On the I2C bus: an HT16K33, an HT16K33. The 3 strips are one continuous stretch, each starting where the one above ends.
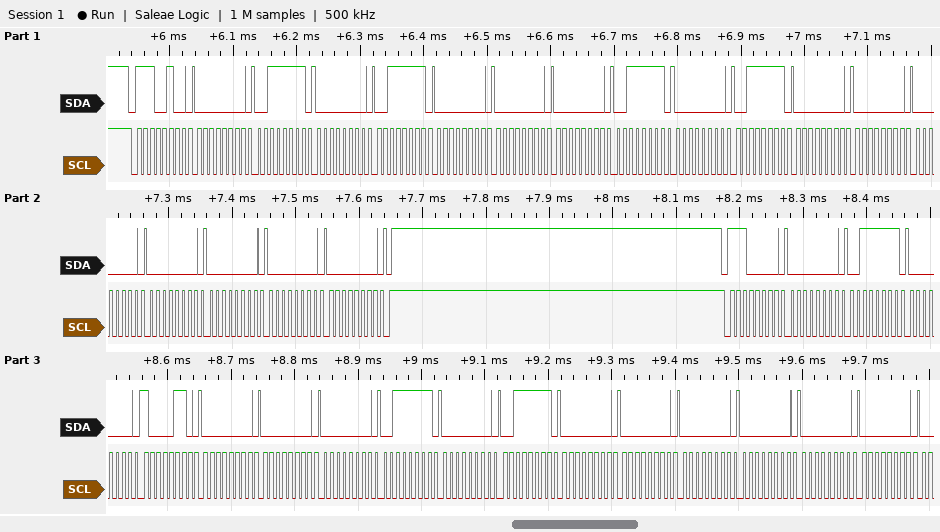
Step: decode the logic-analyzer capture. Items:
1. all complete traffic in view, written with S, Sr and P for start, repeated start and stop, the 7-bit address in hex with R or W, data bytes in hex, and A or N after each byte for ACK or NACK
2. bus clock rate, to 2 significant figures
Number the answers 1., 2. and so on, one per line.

1. S 72W A 00 A 3F A 00 A 3F A 00 A 00 A 00 A 3F A 00 A 3F A 00 A 00 A 00 A 00 A 00 A 00 A 00 A P S 70W A 00 A 3F A 00 A 86 A 00 A 00 A 00 A 3F A 00 A 3F A 00 A 00 A 00 A 00 A 00 A 00 A
2. 100 kHz
